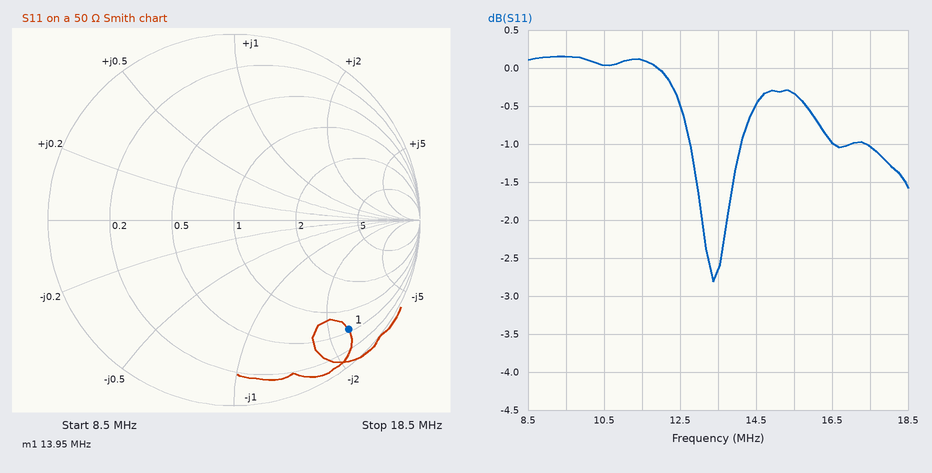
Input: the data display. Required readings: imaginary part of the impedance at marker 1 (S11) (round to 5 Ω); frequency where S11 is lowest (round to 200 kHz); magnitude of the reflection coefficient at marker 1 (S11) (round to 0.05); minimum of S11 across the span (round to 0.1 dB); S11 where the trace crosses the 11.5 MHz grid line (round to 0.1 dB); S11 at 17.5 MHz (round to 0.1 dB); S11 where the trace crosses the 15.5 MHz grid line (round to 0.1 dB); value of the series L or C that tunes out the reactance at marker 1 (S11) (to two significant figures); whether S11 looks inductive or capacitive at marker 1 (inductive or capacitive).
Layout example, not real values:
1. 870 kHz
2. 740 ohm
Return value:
1. -120 Ω
2. 13.4 MHz
3. 0.85
4. -2.8 dB
5. 0.1 dB
6. -1.0 dB
7. -0.3 dB
8. 1.4 µH
9. capacitive
